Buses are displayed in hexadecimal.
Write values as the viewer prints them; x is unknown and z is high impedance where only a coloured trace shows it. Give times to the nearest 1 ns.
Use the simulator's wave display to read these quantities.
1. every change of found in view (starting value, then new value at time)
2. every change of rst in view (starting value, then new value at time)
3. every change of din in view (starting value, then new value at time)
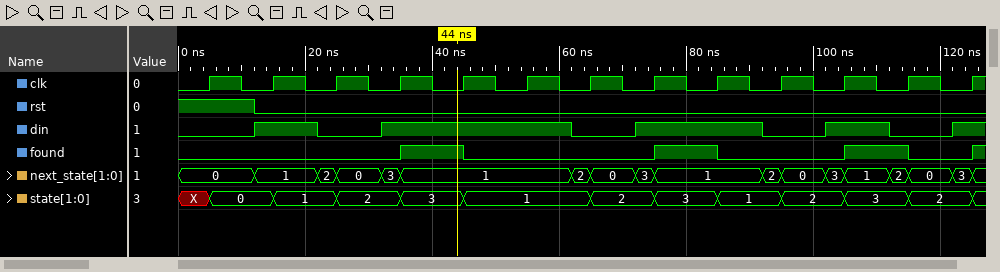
0, 1 at 35 ns, 0 at 45 ns, 1 at 75 ns, 0 at 85 ns, 1 at 105 ns, 0 at 115 ns, 1 at 125 ns
1, 0 at 12 ns
0, 1 at 12 ns, 0 at 22 ns, 1 at 32 ns, 0 at 62 ns, 1 at 72 ns, 0 at 92 ns, 1 at 102 ns, 0 at 112 ns, 1 at 122 ns
